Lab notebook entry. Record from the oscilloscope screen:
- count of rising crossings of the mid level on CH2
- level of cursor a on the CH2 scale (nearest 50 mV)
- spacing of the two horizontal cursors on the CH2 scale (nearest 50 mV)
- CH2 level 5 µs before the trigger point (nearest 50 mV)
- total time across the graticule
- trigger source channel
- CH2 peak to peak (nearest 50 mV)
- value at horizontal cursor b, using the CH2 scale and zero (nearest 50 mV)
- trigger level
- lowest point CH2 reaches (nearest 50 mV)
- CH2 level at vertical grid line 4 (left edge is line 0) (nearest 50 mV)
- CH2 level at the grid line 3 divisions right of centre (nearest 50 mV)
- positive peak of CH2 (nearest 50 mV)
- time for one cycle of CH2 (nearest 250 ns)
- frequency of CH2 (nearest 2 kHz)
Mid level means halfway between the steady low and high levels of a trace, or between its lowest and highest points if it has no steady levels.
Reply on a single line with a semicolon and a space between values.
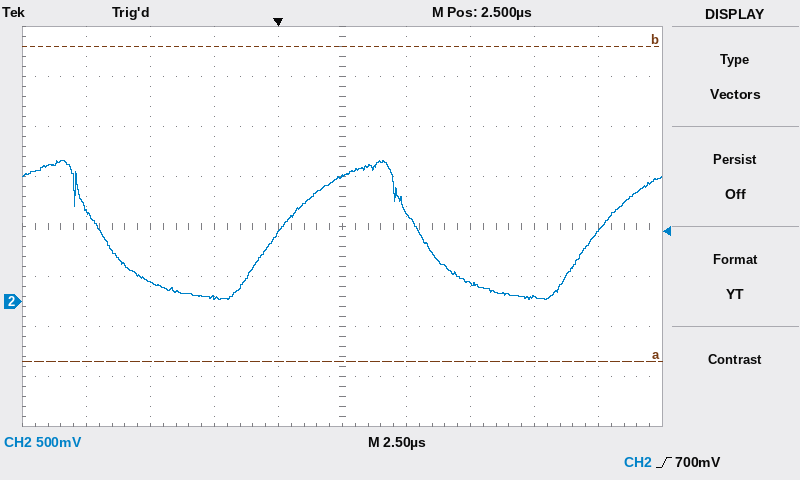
2; -600 mV; 3.15 V; 200 mV; 25 µs; CH2; 1.40 V; 2.55 V; 700 mV; 0 mV; 700 mV; 50 mV; 1.40 V; 12.50 µs; 80 kHz
